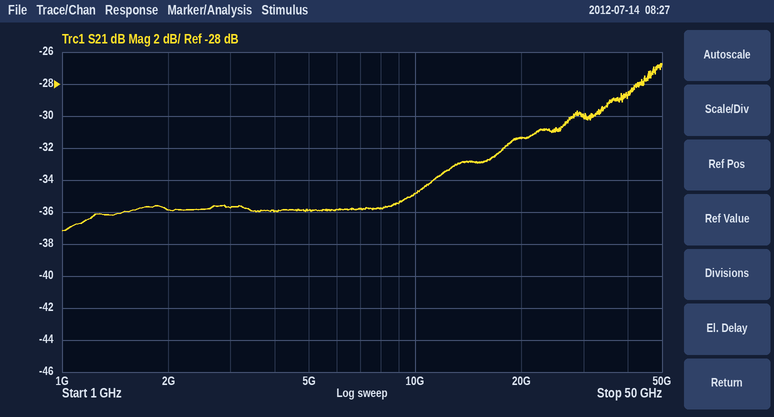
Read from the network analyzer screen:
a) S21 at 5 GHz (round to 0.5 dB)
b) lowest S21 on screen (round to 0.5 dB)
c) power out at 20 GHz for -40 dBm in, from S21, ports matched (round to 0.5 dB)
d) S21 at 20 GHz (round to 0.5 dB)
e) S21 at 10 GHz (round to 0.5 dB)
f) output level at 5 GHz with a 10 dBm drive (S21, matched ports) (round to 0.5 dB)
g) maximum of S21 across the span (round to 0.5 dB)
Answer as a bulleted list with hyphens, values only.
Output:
- -36.0 dB
- -37.0 dB
- -71.5 dBm
- -31.5 dB
- -35.0 dB
- -26.0 dBm
- -26.5 dB
